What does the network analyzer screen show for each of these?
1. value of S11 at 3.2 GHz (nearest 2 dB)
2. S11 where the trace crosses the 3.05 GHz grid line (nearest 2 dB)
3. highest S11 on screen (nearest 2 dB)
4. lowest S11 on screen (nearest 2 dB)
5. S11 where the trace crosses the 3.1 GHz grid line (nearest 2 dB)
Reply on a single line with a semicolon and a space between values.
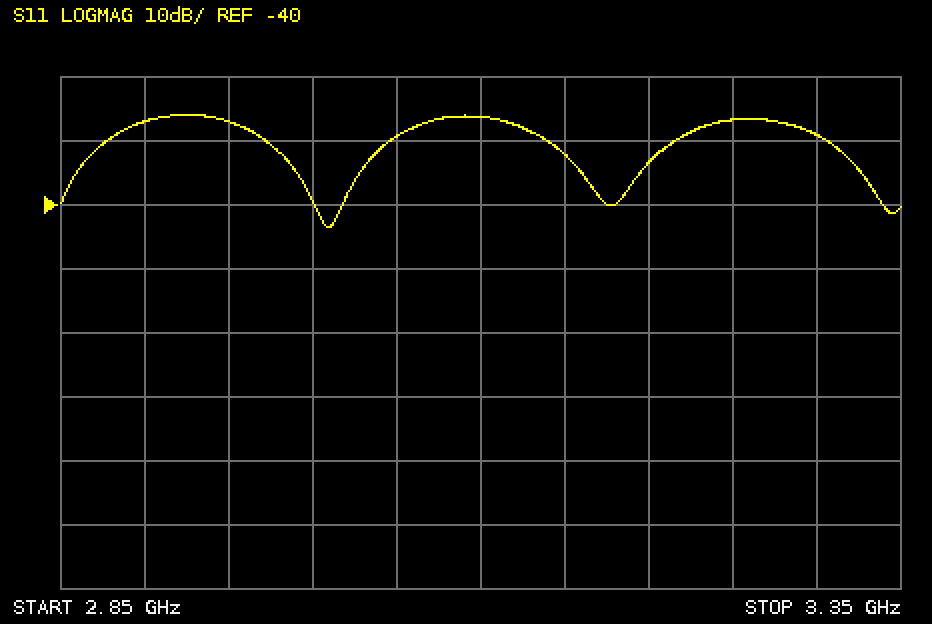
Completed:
-34 dB; -30 dB; -26 dB; -44 dB; -26 dB
